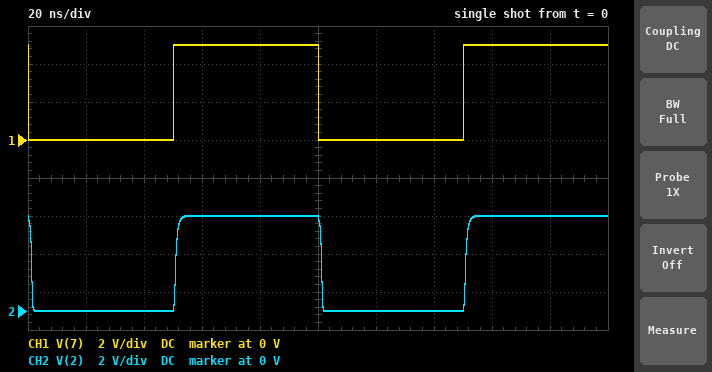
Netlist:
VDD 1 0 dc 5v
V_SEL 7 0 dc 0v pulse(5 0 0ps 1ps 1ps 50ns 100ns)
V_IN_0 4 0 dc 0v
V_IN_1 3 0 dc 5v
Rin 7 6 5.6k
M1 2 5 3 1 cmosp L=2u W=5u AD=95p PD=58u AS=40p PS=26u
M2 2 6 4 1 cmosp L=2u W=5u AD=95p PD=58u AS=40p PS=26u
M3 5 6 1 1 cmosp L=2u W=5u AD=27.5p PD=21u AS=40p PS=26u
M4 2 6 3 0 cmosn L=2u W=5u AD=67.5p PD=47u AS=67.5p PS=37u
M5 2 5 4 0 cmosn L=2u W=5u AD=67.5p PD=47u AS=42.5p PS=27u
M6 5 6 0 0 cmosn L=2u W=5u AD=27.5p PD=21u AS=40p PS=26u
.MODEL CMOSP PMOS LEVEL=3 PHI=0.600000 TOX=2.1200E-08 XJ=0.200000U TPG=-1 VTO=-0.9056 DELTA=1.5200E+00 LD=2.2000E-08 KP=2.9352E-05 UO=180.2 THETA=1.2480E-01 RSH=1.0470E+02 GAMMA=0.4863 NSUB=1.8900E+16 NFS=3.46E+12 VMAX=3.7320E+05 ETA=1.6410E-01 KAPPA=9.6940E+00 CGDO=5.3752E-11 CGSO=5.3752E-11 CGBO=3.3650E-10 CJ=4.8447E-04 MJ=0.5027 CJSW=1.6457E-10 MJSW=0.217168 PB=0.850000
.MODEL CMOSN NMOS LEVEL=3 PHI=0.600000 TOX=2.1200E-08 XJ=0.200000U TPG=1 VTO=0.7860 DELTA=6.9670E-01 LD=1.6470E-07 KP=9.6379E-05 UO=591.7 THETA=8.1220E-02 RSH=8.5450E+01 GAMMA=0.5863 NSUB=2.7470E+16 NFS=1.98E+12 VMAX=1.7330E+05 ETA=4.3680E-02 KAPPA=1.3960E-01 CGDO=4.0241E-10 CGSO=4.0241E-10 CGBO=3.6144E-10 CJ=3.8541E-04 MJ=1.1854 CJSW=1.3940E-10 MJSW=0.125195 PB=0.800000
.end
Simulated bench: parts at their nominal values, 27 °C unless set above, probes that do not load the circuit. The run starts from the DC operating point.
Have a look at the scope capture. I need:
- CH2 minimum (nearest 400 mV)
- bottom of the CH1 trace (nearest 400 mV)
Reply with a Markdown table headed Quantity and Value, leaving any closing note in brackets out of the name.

| Quantity | Value |
|---|---|
| CH2 minimum | 0 V |
| bottom of the CH1 trace | 0 V |
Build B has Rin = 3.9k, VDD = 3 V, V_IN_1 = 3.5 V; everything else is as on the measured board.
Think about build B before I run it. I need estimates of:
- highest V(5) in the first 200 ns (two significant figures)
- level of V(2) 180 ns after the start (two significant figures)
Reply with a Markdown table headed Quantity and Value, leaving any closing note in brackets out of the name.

| Quantity | Value |
|---|---|
| highest V(5) in the first 200 ns | 3.3 V |
| level of V(2) 180 ns after the start | 3.5 V |
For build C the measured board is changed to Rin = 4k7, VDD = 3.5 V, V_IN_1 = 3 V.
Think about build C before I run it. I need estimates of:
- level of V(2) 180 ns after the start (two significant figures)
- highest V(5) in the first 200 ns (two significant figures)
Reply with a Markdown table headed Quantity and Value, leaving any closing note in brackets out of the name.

| Quantity | Value |
|---|---|
| level of V(2) 180 ns after the start | 3.0 V |
| highest V(5) in the first 200 ns | 3.7 V |
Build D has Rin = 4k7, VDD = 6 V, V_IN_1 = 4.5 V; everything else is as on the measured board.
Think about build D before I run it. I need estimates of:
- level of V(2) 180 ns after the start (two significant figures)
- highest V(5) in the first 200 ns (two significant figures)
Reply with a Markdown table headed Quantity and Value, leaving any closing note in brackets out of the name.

| Quantity | Value |
|---|---|
| level of V(2) 180 ns after the start | 4.5 V |
| highest V(5) in the first 200 ns | 6.2 V |
